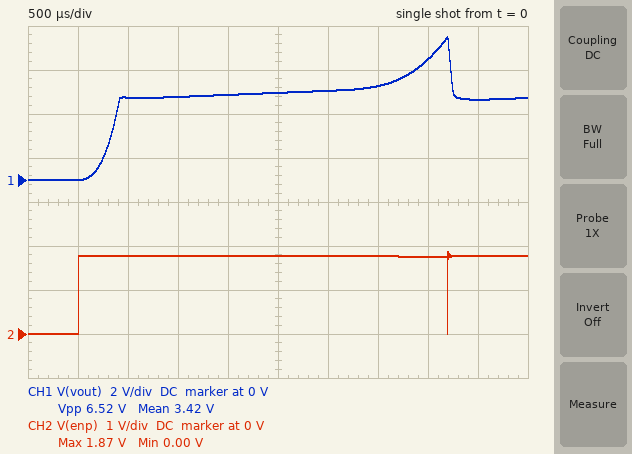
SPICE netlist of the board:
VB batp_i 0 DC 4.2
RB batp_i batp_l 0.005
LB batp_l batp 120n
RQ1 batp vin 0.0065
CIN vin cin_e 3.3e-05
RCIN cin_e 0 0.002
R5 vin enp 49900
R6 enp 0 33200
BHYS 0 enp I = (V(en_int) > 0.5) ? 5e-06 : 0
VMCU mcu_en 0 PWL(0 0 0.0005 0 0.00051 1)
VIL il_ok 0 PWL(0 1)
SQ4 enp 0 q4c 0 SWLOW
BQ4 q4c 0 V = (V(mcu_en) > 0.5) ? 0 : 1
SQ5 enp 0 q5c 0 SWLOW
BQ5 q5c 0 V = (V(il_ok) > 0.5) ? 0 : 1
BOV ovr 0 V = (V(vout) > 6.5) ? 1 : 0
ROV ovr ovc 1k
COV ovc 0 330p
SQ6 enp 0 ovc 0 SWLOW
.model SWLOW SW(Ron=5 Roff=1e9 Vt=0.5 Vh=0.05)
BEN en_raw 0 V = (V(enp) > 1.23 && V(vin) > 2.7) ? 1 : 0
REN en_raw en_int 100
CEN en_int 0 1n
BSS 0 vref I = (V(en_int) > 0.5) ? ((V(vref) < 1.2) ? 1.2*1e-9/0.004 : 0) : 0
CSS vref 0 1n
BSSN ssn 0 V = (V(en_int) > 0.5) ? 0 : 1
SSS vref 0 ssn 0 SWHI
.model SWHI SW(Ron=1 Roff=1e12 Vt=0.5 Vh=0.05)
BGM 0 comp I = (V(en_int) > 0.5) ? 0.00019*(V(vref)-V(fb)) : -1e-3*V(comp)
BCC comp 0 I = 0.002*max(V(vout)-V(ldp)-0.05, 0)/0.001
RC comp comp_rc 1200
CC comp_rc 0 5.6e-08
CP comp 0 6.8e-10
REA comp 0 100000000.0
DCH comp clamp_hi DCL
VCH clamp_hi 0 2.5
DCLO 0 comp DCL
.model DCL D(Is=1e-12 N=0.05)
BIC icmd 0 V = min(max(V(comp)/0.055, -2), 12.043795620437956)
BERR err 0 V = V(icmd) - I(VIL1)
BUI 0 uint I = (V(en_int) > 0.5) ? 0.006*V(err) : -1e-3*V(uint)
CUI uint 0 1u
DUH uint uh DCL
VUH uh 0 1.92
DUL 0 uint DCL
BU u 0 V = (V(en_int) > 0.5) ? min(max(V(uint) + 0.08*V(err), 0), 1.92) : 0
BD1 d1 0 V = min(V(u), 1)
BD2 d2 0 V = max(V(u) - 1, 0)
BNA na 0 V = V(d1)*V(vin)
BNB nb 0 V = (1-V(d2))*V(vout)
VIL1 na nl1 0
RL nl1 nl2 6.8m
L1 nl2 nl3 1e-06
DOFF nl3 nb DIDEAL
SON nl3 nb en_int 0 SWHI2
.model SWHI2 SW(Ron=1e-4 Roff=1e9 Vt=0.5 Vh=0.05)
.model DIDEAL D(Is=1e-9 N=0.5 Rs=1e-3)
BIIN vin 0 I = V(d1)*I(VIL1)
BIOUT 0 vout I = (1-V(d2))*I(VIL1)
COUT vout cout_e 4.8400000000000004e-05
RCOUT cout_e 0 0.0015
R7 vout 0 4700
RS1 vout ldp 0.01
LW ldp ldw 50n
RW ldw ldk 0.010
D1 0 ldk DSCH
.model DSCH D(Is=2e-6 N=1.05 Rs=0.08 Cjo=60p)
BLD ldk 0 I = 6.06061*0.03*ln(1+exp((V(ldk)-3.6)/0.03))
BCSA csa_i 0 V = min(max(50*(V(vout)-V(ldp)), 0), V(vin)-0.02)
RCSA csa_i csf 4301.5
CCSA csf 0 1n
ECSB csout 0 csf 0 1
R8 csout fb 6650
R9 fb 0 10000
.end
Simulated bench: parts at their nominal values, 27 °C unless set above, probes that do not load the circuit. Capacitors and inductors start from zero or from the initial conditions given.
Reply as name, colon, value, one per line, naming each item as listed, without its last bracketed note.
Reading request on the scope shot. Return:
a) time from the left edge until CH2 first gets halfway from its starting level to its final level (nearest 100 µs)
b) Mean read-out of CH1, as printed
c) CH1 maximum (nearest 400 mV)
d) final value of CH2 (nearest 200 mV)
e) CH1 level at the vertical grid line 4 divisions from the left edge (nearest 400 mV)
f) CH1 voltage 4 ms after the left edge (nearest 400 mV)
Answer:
time from the left edge until CH2 first gets halfway from its starting level to its final level: 500 µs
Mean read-out of CH1, as printed: 3.42 V
CH1 maximum: 6.4 V
final value of CH2: 1.8 V
CH1 level at the vertical grid line 4 divisions from the left edge: 4.0 V
CH1 voltage 4 ms after the left edge: 5.6 V
